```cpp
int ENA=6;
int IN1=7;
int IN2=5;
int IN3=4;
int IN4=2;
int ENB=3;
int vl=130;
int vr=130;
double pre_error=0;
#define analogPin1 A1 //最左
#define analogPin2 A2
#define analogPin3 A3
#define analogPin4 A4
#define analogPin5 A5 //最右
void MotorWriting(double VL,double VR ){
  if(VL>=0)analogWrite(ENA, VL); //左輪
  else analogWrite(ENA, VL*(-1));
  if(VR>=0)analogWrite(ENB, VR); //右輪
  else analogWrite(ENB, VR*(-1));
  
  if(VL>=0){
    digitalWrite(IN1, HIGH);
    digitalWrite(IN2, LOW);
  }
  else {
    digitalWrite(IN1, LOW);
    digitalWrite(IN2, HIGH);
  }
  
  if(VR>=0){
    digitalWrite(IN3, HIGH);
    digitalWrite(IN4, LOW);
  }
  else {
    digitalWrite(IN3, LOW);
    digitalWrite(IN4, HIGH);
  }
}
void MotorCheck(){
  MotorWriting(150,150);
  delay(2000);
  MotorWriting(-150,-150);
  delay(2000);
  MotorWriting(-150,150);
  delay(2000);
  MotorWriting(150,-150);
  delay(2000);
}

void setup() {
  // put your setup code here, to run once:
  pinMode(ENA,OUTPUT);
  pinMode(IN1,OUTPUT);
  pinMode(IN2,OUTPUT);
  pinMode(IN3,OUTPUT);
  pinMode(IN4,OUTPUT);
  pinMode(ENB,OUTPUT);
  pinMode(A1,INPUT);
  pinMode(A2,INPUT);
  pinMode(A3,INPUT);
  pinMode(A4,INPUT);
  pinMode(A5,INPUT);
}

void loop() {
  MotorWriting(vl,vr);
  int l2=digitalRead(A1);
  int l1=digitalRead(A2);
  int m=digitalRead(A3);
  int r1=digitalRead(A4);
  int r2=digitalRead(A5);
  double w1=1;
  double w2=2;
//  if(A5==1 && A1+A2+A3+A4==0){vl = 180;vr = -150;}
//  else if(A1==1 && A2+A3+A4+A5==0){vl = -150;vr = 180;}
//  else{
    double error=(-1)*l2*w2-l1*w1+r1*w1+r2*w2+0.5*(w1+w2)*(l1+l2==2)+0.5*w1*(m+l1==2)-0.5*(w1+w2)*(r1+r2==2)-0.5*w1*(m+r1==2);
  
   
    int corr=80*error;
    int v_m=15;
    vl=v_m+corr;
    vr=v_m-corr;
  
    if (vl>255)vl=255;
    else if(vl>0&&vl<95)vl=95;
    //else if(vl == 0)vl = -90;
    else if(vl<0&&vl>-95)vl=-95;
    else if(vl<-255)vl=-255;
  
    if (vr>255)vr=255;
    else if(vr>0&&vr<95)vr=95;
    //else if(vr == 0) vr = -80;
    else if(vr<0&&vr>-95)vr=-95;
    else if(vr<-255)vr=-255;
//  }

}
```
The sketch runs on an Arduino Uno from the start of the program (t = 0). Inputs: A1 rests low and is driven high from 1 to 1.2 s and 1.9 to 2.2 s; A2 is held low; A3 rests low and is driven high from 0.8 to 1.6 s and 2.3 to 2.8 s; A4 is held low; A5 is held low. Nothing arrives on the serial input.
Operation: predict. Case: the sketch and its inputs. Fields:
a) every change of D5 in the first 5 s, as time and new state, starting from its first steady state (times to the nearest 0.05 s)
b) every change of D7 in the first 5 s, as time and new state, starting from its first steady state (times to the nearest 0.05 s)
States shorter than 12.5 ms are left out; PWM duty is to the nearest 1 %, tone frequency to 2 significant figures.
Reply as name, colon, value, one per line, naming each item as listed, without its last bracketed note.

every change of D5 in the first 5 s, as time and new state, starting from its first steady state: 0 s low; 1 s high; 1.2 s low; 1.9 s high; 2.2 s low
every change of D7 in the first 5 s, as time and new state, starting from its first steady state: 0 s high; 1 s low; 1.2 s high; 1.9 s low; 2.2 s high
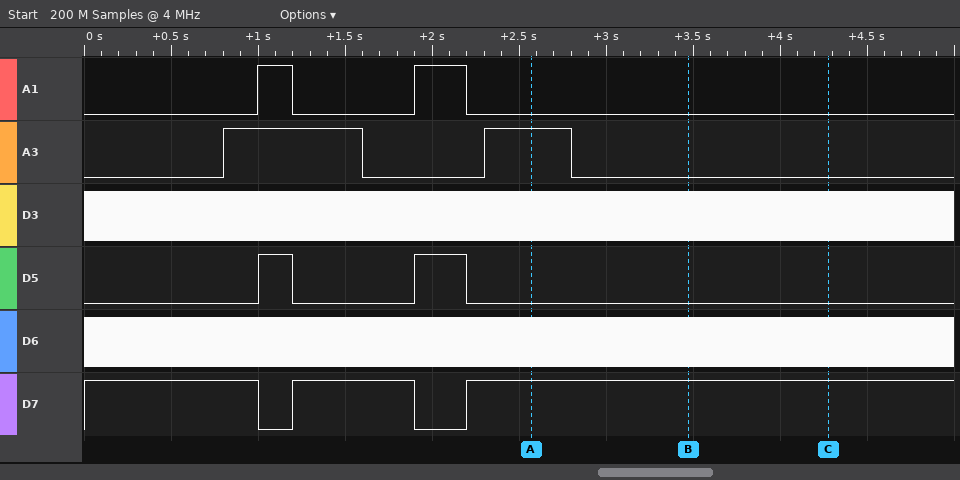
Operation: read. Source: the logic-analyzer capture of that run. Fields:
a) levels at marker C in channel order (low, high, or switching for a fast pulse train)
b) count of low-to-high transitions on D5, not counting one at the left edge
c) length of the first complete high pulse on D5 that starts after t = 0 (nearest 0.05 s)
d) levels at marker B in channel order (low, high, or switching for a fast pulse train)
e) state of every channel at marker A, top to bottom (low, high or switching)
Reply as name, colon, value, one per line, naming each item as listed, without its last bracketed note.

levels at marker C in channel order: A1 low, A3 low, D3 switching, D5 low, D6 switching, D7 high
count of low-to-high transitions on D5, not counting one at the left edge: 2
length of the first complete high pulse on D5 that starts after t = 0: 0.20 s
levels at marker B in channel order: A1 low, A3 low, D3 switching, D5 low, D6 switching, D7 high
state of every channel at marker A, top to bottom: A1 low, A3 high, D3 switching, D5 low, D6 switching, D7 high
